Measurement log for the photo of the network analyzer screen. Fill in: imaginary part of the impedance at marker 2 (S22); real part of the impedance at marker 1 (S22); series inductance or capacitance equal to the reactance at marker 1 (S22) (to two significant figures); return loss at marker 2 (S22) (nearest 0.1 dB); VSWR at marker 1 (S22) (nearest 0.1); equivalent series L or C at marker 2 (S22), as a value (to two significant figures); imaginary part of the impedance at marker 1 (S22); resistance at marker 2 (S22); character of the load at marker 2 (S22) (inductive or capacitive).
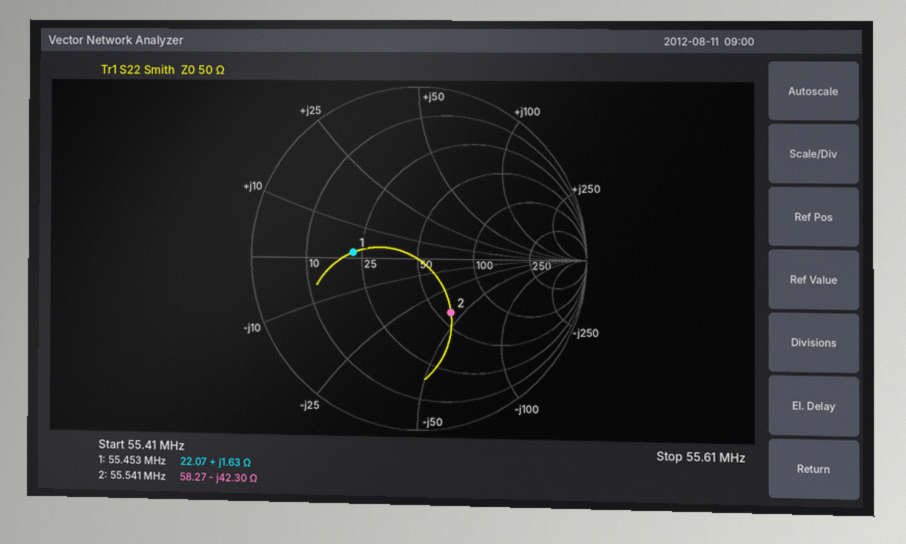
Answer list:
-42.30 Ω
22.07 Ω
4.7 nH
8.6 dB
2.3
68 pF
+1.63 Ω
58.27 Ω
capacitive
